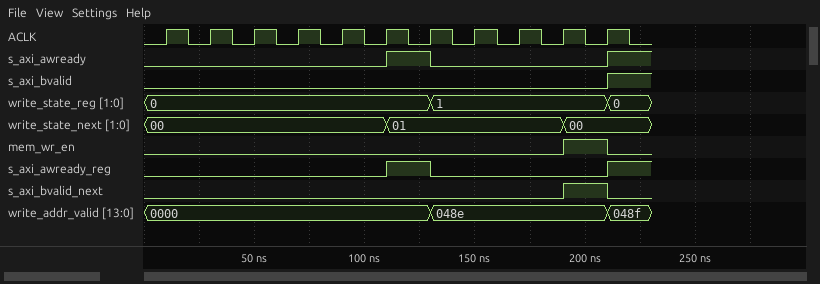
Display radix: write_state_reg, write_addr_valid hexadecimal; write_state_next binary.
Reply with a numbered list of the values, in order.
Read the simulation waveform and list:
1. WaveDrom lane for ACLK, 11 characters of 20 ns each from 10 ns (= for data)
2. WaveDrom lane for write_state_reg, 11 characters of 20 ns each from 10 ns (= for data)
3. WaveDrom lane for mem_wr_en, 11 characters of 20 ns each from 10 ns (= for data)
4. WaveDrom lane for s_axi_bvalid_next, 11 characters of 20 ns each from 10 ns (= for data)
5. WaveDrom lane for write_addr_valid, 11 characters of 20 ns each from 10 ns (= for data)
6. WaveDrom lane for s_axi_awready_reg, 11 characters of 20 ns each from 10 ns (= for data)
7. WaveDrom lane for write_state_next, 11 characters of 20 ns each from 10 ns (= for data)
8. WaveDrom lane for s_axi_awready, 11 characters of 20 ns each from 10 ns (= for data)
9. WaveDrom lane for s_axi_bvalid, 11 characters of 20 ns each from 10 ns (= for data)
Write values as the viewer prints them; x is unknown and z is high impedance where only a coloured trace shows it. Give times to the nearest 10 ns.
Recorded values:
1. {name: 'ACLK', wave: 'p..........'}
2. {name: 'write_state_reg', wave: '=.....=...=', data: '0 1 0'}
3. {name: 'mem_wr_en', wave: '0........10'}
4. {name: 's_axi_bvalid_next', wave: '0........10'}
5. {name: 'write_addr_valid', wave: '=.....=...=', data: '0000 048e 048f'}
6. {name: 's_axi_awready_reg', wave: '0....10...1'}
7. {name: 'write_state_next', wave: '=....=...=.', data: '00 01 00'}
8. {name: 's_axi_awready', wave: '0....10...1'}
9. {name: 's_axi_bvalid', wave: '0.........1'}
